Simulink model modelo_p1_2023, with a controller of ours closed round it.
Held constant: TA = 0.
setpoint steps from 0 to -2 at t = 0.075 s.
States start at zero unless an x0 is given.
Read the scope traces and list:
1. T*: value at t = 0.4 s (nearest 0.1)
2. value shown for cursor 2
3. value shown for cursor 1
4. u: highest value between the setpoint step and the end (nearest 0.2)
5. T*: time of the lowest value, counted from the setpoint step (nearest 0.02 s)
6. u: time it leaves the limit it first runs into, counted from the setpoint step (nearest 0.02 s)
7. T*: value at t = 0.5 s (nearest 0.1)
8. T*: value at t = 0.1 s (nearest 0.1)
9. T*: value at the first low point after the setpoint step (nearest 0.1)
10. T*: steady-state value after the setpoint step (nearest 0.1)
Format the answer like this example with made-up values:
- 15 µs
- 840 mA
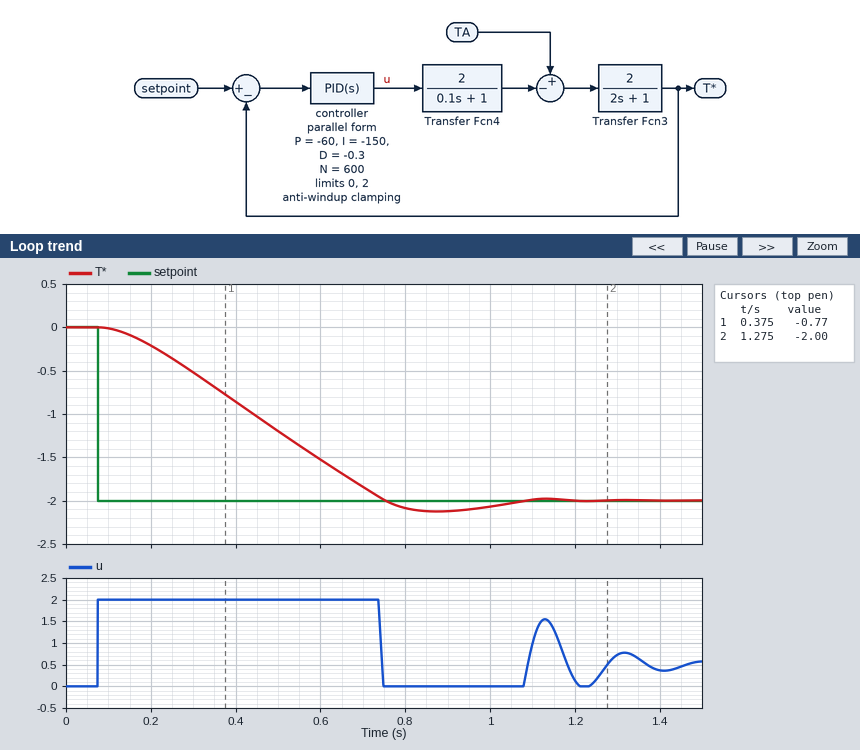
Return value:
- -0.9
- -2.00
- -0.77
- 2.0
- 0.80 s
- 0.66 s
- -1.2
- 0.0
- -2.1
- -2.0
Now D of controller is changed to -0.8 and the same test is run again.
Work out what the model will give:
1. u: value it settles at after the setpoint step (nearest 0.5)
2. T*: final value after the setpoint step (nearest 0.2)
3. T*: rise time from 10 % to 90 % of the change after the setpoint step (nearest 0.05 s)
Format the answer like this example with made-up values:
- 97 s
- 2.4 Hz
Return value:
- 0.5
- -2.0
- 0.50 s
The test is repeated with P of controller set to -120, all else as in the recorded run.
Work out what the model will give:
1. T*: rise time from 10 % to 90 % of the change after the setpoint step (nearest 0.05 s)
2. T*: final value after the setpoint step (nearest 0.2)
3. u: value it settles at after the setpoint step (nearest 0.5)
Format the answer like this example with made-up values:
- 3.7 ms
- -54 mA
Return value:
- 0.50 s
- -2.0
- 0.5
